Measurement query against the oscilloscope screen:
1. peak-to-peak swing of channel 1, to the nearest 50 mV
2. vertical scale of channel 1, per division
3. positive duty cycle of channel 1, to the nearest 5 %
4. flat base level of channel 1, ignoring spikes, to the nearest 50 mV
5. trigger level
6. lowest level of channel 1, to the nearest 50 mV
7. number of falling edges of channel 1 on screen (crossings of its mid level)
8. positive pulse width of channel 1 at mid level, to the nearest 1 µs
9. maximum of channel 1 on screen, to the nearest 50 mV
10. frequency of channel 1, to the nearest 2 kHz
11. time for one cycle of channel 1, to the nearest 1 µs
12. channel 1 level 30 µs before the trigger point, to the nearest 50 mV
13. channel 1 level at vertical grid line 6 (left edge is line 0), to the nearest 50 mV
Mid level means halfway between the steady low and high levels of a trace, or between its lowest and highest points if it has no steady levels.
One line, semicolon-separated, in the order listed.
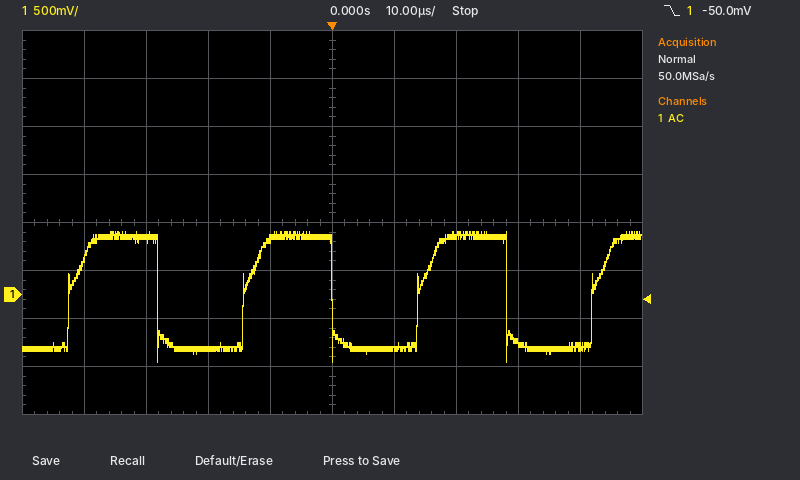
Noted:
1.35 V; 500 mV; 50 %; -550 mV; -50.0 mV; -700 mV; 3; 14 µs; 650 mV; 36 kHz; 28 µs; 600 mV; -550 mV
